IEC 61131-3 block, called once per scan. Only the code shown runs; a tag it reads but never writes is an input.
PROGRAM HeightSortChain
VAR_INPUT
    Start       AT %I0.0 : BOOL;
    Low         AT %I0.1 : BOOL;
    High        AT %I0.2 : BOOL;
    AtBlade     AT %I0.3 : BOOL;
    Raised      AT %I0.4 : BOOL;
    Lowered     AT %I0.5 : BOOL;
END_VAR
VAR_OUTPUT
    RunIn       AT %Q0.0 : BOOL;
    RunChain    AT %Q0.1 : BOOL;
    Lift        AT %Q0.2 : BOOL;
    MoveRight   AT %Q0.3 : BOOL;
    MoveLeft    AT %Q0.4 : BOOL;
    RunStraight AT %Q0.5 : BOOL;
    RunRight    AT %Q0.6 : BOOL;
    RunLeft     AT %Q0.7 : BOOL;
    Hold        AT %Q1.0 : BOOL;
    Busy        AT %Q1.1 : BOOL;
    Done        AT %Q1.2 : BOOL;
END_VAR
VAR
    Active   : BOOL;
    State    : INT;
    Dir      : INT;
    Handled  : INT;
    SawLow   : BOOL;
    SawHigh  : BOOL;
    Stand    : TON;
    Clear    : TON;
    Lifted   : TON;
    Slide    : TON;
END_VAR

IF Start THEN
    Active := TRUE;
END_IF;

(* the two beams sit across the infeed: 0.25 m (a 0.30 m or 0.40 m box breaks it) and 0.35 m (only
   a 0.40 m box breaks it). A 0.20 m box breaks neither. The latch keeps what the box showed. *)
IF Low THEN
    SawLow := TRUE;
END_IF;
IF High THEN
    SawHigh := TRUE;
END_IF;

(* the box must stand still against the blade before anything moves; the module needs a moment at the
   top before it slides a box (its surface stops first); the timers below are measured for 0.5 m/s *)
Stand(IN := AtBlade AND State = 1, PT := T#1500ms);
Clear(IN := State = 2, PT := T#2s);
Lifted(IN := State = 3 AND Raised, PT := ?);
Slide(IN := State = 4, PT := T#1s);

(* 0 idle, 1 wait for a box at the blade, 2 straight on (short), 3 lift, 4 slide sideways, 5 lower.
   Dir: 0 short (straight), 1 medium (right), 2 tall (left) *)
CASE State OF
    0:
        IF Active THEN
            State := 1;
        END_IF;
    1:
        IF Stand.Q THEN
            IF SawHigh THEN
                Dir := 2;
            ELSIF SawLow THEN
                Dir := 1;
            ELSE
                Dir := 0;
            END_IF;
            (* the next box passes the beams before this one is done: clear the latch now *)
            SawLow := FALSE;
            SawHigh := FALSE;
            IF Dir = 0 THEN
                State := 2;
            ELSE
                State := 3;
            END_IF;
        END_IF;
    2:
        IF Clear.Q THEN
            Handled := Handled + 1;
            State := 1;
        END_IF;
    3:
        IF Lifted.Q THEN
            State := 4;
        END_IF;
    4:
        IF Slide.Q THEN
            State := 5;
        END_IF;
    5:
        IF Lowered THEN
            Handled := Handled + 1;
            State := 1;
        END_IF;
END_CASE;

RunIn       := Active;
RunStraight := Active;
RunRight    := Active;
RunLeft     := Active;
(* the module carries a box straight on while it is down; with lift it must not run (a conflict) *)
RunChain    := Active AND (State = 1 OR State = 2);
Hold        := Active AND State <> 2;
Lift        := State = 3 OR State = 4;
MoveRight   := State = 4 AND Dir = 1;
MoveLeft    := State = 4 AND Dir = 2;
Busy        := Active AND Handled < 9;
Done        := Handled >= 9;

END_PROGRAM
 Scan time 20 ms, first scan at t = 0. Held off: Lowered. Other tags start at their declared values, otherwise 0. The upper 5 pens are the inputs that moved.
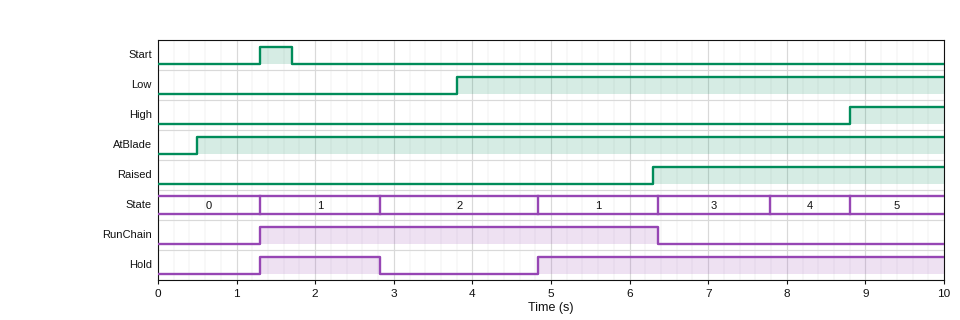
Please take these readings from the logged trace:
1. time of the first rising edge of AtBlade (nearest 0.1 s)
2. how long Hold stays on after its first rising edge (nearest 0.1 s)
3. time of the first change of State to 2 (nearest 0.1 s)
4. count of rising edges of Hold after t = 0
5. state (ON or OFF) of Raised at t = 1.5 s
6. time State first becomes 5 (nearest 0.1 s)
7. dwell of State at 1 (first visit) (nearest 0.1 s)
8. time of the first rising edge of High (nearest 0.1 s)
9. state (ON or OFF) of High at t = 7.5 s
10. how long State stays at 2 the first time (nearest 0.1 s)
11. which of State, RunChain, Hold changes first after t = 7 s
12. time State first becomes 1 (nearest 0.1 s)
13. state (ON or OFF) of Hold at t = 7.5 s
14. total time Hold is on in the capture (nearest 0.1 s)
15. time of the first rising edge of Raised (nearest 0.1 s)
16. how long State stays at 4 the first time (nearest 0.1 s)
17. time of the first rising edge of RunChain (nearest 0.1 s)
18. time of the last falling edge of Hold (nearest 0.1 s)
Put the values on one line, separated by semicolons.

0.5 s; 1.5 s; 2.8 s; 2; OFF; 8.8 s; 1.5 s; 8.8 s; OFF; 2.0 s; State; 1.3 s; ON; 6.7 s; 6.3 s; 1.0 s; 1.3 s; 2.8 s
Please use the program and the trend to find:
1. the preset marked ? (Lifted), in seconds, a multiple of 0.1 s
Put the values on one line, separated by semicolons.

1.4 s
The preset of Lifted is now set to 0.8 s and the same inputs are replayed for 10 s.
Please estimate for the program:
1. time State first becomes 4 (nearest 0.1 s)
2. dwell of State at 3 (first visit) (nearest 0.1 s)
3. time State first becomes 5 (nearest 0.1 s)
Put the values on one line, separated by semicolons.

7.2 s; 0.8 s; 8.2 s
